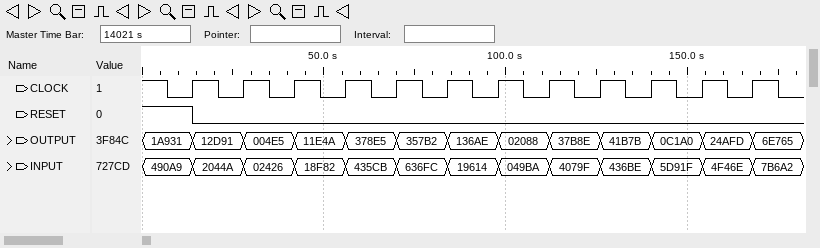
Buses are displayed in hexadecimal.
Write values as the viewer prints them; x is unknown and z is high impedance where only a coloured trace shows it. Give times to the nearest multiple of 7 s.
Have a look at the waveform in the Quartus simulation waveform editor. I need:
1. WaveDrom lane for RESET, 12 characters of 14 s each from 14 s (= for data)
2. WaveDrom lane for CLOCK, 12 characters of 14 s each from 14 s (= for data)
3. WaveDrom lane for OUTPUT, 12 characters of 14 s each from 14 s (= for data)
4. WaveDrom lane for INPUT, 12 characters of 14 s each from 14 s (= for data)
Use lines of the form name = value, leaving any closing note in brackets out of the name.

WaveDrom lane for RESET, 12 characters of 14 s each from 14 s = {name: 'RESET', wave: '0...........'}
WaveDrom lane for CLOCK, 12 characters of 14 s each from 14 s = {name: 'CLOCK', wave: 'p...........'}
WaveDrom lane for OUTPUT, 12 characters of 14 s each from 14 s = {name: 'OUTPUT', wave: '============', data: '12D91 004E5 11E4A 378E5 357B2 136AE 02088 37B8E 41B7B 0C1A0 24AFD 6E765'}
WaveDrom lane for INPUT, 12 characters of 14 s each from 14 s = {name: 'INPUT', wave: '============', data: '2044A 02426 18F82 435CB 636FC 19614 049BA 4079F 436BE 5D91F 4F46E 7B6A2'}
